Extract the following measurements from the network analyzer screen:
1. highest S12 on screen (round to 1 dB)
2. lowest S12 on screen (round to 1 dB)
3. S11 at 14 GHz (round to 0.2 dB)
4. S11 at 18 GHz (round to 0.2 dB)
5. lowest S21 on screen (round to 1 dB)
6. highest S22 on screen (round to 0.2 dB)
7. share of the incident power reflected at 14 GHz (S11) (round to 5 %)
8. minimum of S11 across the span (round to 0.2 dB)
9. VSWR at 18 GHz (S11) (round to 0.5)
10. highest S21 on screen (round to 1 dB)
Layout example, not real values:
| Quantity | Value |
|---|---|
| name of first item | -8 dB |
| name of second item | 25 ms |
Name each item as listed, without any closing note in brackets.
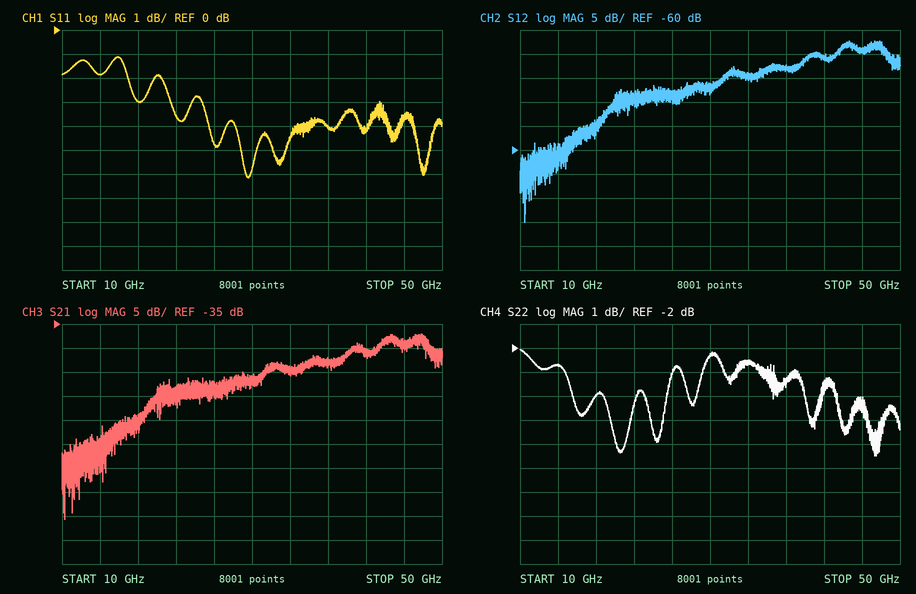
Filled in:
| Quantity | Value |
|---|---|
| highest S12 on screen | -37 dB |
| lowest S12 on screen | -75 dB |
| S11 at 14 GHz | -1.8 dB |
| S11 at 18 GHz | -3.0 dB |
| lowest S21 on screen | -76 dB |
| highest S22 on screen | -2.0 dB |
| share of the incident power reflected at 14 GHz (S11) | 65 % |
| minimum of S11 across the span | -6.2 dB |
| VSWR at 18 GHz (S11) | 6.0 |
| highest S21 on screen | -37 dB |
